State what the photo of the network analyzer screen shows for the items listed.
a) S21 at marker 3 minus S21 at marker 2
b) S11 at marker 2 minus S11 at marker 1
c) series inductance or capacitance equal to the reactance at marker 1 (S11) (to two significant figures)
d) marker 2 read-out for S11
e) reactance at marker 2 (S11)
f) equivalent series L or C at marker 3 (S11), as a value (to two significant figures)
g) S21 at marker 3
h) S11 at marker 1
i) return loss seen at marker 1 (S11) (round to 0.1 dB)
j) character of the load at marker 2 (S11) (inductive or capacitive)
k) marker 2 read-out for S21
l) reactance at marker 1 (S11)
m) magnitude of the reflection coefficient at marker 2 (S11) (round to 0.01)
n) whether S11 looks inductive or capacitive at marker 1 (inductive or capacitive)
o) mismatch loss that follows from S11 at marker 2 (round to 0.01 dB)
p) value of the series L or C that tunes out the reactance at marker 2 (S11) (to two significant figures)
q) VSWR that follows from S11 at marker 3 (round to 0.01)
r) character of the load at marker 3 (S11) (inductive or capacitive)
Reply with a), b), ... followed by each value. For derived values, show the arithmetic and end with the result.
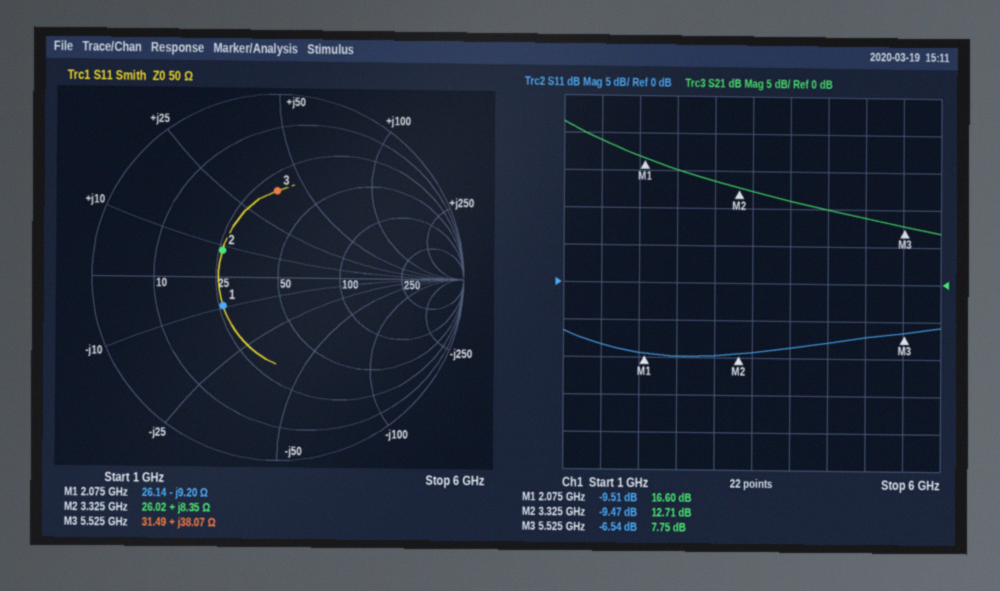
a) 7.75 − (12.71) = -4.96 dB
b) -9.47 − (-9.51) = 0.04 dB
c) C = 1/(2π × 2.075 GHz × 9.2 Ω) ≈ 8.3 pF
d) -9.47 dB
e) +8.35 Ω
f) L = 38.07 Ω/(2π × 5.525 GHz) ≈ 1.1 nH
g) 7.75 dB
h) -9.51 dB
i) 9.5 dB
j) inductive
k) 12.71 dB
l) -9.20 Ω
m) 0.33
n) capacitive
o) −10 log10(1 − 10^(-9.47/10)) ≈ 0.52 dB
p) C = 1/(2π × 3.325 GHz × 8.35 Ω) ≈ 5.7 pF
q) (1 + 0.4710)/(1 − 0.4710) ≈ 2.78
r) inductive
